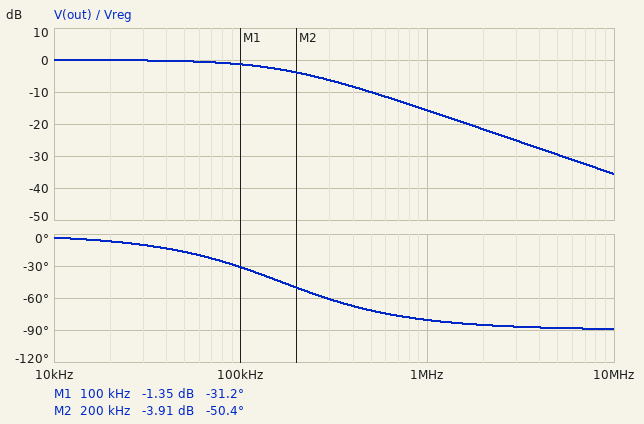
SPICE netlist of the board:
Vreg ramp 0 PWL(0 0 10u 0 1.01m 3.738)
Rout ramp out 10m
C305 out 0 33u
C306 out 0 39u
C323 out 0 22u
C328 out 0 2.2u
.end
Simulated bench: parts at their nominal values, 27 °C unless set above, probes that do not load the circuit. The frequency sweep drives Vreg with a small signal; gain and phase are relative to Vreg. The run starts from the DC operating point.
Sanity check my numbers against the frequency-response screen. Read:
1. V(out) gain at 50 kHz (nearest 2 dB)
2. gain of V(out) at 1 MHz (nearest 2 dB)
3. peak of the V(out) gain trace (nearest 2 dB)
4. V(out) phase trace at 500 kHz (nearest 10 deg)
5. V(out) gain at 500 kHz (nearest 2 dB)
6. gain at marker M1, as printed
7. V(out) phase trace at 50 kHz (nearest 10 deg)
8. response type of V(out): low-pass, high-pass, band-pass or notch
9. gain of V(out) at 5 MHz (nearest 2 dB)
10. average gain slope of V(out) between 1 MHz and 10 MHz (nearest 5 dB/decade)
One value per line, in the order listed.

0 dB
-16 dB
0 dB
-70 deg
-10 dB
-1.35 dB
-20 deg
low-pass
-30 dB
-20 dB/decade
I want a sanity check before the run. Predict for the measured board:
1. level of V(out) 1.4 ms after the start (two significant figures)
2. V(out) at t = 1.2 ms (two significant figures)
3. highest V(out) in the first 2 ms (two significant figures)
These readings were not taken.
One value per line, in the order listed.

3.7 V
3.7 V
3.7 V
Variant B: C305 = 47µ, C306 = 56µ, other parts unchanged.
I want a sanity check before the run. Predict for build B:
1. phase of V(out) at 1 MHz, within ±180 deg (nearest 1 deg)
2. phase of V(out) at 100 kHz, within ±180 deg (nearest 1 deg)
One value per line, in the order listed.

-83 deg
-39 deg
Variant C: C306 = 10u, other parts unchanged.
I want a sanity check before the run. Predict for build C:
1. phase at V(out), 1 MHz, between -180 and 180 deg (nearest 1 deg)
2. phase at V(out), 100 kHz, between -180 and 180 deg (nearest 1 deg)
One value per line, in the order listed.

-77 deg
-23 deg
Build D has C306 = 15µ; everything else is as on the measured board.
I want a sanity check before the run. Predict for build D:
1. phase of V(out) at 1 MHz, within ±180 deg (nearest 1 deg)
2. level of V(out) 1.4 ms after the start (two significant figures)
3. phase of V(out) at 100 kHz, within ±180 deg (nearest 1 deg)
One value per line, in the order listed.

-78 deg
3.7 V
-24 deg
